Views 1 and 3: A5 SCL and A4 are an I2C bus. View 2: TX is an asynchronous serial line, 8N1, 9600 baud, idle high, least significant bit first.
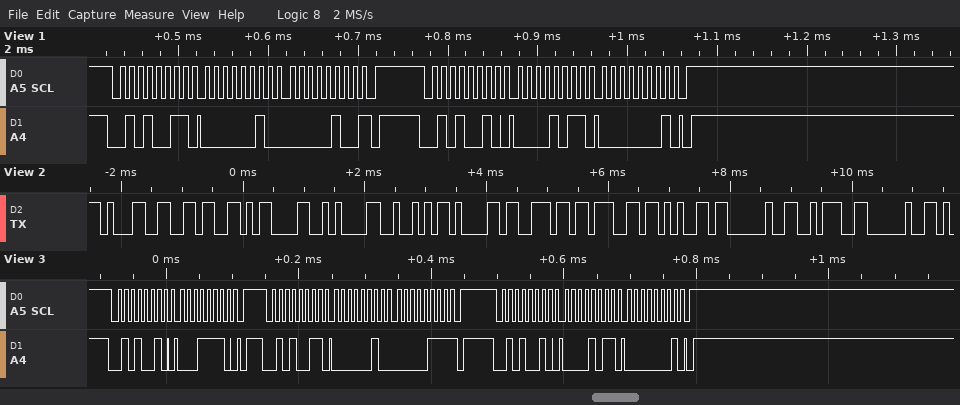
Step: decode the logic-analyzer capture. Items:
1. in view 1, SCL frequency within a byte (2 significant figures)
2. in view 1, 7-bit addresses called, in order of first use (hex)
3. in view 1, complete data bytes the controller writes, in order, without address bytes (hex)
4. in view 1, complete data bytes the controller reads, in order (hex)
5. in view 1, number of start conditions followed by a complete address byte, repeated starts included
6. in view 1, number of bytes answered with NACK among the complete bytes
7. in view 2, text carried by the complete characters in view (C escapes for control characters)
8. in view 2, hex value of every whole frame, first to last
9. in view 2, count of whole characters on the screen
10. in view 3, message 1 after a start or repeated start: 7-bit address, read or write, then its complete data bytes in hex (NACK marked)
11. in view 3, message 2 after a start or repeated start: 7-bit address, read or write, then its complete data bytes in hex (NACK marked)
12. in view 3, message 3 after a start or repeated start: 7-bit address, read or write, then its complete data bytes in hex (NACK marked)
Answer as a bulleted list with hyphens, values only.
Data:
- 100 kHz
- 0x29
- 0B 01
- 02 04
- 2
- 1
- "16\r\nRange : "
- 31 36 0D 0A 52 61 6E 67 65 20 3A 20
- 12
- 0x29 write: 1E
- 0x29 read: 02 07 NACK
- 0x29 write: 0B 01
